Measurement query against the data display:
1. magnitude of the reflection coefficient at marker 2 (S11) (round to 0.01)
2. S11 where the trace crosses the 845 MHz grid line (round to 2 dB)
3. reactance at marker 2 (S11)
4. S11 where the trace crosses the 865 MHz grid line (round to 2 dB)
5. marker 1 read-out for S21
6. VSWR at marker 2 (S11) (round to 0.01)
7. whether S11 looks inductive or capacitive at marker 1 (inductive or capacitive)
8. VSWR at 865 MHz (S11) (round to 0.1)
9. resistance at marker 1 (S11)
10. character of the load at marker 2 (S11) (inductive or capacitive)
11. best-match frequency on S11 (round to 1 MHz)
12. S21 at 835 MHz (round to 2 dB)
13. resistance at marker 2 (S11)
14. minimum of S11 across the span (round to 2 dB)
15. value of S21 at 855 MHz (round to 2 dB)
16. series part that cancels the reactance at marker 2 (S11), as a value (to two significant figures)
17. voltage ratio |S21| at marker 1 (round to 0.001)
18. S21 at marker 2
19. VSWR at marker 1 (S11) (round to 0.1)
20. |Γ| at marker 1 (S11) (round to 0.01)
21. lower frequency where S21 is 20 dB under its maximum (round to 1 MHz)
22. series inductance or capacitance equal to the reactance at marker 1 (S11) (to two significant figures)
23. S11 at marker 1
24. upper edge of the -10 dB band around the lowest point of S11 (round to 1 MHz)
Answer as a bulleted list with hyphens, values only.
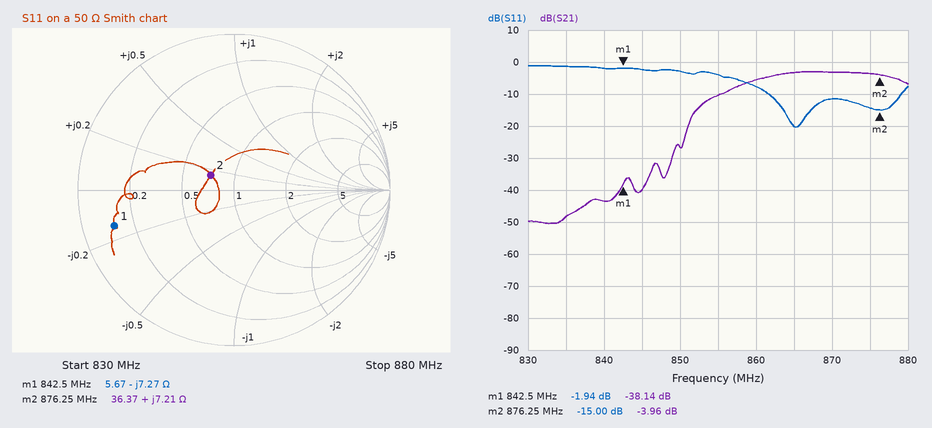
- 0.18
- -2 dB
- +7.21 Ω
- -20 dB
- -38.14 dB
- 1.43
- capacitive
- 1.2
- 5.67 Ω
- inductive
- 865 MHz
- -48 dB
- 36.37 Ω
- -20 dB
- -10 dB
- 25 pF
- 0.012
- -3.96 dB
- 9.0
- 0.80
- 851 MHz
- 26 pF
- -1.94 dB
- 879 MHz
